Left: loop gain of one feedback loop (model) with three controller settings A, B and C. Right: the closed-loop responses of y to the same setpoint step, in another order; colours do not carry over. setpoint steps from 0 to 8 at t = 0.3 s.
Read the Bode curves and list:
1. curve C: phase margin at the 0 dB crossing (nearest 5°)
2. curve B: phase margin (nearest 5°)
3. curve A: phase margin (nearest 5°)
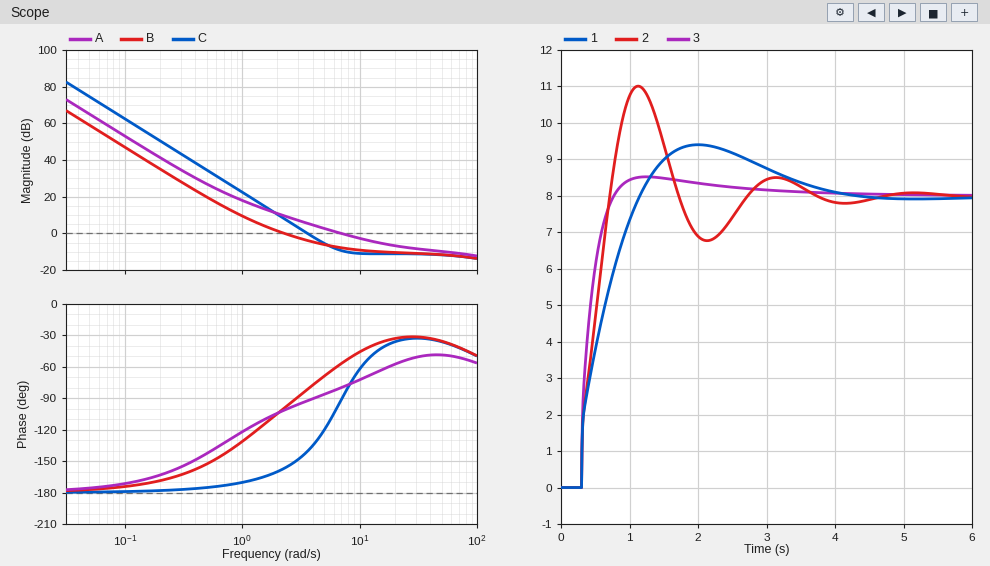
40°
80°
100°
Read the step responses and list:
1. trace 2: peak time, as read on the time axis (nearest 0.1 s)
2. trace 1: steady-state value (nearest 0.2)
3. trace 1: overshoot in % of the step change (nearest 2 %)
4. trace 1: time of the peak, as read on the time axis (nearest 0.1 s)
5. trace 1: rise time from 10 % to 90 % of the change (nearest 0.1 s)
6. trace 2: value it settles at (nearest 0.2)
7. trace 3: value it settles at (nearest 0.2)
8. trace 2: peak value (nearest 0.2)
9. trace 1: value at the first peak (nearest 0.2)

1.1 s
8.0
18 %
2.0 s
0.7 s
8.0
8.0
11.0
9.4
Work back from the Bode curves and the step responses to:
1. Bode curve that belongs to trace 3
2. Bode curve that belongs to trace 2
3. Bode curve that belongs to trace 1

A
C
B
